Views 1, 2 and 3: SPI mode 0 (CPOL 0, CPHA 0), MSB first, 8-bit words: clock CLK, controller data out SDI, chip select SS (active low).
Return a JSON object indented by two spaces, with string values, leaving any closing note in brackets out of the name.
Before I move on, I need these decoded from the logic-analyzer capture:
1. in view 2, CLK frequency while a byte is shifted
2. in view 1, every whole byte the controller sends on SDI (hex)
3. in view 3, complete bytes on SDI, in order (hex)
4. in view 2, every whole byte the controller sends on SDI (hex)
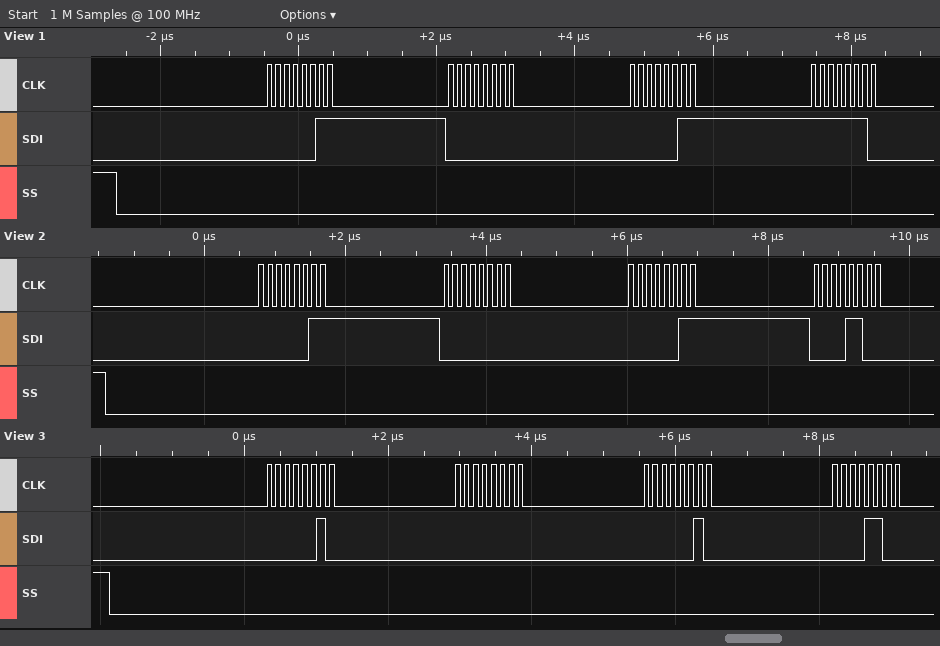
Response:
{
  "in view 2, CLK frequency while a byte is shifted": "8 MHz",
  "in view 1, every whole byte the controller sends on SDI": "03 00 03 FE",
  "in view 3, complete bytes on SDI, in order": "02 00 02 0C",
  "in view 2, every whole byte the controller sends on SDI": "03 00 03 0C"
}
